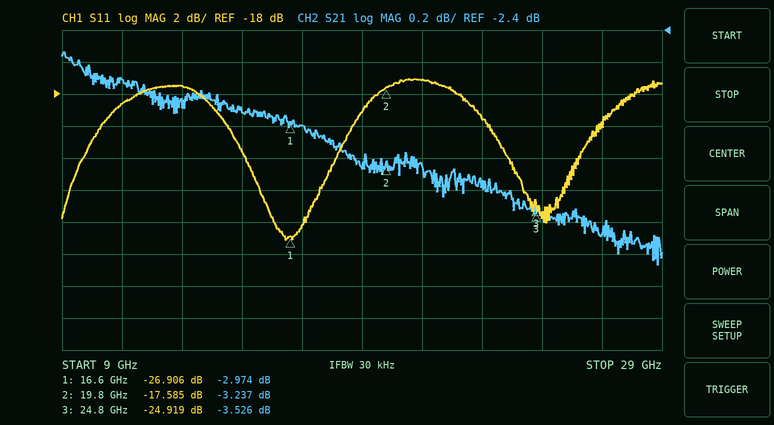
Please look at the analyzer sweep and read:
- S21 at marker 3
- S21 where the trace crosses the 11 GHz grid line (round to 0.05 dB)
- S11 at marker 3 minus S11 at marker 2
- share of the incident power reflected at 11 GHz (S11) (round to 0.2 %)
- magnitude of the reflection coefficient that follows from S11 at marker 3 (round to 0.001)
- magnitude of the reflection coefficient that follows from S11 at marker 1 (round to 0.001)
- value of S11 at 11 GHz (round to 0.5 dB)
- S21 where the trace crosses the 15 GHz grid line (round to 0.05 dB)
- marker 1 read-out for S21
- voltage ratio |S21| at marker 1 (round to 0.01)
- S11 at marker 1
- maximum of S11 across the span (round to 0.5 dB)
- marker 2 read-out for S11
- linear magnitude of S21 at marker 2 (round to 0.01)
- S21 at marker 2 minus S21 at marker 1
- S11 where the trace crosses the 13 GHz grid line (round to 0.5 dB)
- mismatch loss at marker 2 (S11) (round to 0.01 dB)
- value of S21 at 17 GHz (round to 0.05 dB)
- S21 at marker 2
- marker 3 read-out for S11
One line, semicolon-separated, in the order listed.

-3.526 dB; -2.70 dB; -7.334 dB; 1.4 %; 0.057; 0.045; -18.5 dB; -2.90 dB; -2.974 dB; 0.71; -26.906 dB; -17.0 dB; -17.585 dB; 0.69; -0.263 dB; -17.5 dB; 0.08 dB; -3.00 dB; -3.237 dB; -24.919 dB
